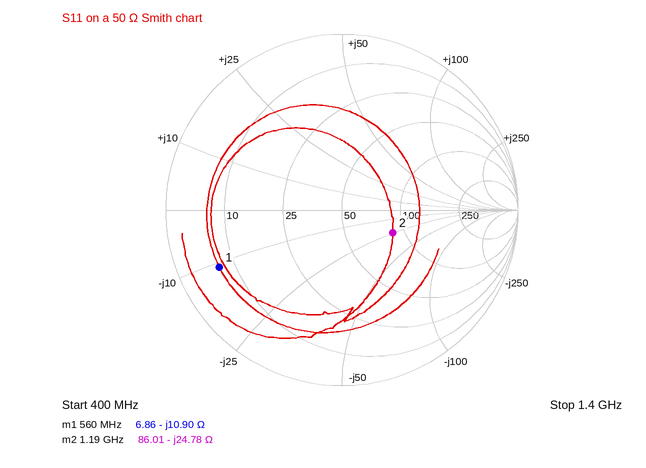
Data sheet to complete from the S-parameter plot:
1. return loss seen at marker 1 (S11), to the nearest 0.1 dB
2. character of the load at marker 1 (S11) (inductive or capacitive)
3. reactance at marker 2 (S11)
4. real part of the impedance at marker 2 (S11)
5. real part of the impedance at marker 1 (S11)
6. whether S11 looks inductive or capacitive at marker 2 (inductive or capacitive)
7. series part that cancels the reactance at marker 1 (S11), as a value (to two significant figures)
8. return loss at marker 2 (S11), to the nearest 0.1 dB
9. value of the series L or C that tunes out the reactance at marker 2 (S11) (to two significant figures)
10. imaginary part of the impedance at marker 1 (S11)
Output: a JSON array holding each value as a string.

["2.3 dB", "capacitive", "-24.78 Ω", "86.01 Ω", "6.86 Ω", "capacitive", "3.1 nH", "10.0 dB", "3.3 nH", "-10.90 Ω"]
